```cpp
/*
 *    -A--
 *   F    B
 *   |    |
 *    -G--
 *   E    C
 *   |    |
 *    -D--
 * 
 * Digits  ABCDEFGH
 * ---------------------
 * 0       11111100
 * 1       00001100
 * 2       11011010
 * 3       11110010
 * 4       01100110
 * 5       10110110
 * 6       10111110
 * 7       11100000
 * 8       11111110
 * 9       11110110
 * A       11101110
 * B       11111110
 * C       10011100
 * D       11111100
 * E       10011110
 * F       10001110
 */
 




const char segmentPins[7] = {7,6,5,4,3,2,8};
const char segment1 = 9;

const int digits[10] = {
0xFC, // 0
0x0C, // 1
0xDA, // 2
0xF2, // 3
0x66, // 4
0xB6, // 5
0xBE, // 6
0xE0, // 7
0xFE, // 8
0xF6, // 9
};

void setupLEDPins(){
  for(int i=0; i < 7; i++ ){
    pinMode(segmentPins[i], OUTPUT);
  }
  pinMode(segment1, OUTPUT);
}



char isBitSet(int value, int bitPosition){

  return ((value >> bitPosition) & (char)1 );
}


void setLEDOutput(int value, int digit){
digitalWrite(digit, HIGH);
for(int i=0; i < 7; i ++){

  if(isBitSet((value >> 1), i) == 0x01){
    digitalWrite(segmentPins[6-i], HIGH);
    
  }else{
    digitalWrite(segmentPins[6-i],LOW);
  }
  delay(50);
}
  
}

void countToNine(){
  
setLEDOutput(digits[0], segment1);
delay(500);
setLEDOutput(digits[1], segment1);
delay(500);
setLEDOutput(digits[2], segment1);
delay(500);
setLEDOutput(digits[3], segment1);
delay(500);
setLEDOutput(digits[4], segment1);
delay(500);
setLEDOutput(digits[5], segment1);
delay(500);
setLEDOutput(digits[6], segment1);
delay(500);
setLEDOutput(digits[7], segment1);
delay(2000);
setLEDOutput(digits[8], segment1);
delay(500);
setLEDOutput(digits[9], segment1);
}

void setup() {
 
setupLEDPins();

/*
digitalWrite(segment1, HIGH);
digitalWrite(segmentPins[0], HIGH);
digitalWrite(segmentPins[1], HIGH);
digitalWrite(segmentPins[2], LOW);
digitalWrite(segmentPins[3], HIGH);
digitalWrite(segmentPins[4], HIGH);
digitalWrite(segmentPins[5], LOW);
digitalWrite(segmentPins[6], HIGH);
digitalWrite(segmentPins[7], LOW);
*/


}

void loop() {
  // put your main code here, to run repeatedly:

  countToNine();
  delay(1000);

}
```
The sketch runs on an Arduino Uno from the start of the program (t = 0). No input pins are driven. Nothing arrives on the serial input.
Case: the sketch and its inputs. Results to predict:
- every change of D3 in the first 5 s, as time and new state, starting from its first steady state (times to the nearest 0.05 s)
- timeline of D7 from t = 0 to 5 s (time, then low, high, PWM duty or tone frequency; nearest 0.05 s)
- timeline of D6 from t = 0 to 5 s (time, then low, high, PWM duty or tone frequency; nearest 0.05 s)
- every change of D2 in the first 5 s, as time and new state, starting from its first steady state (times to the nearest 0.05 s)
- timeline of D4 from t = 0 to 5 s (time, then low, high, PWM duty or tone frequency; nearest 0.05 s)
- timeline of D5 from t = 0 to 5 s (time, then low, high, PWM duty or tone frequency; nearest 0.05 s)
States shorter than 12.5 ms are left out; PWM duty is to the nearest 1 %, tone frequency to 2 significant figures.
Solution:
0 s low; 0.1 s high; 2.65 s low
0 s low; 0.3 s high; 1.15 s low; 2 s high; 3.7 s low; 4.55 s high
0 s low; 0.25 s high; 1.1 s low; 1.95 s high; 4.5 s low
0 s low; 0.05 s high; 1.75 s low; 3.45 s high
0 s low; 0.15 s high; 1 s low; 1.85 s high; 3.55 s low; 4.4 s high
0 s low; 0.2 s high; 1.05 s low; 2.75 s high
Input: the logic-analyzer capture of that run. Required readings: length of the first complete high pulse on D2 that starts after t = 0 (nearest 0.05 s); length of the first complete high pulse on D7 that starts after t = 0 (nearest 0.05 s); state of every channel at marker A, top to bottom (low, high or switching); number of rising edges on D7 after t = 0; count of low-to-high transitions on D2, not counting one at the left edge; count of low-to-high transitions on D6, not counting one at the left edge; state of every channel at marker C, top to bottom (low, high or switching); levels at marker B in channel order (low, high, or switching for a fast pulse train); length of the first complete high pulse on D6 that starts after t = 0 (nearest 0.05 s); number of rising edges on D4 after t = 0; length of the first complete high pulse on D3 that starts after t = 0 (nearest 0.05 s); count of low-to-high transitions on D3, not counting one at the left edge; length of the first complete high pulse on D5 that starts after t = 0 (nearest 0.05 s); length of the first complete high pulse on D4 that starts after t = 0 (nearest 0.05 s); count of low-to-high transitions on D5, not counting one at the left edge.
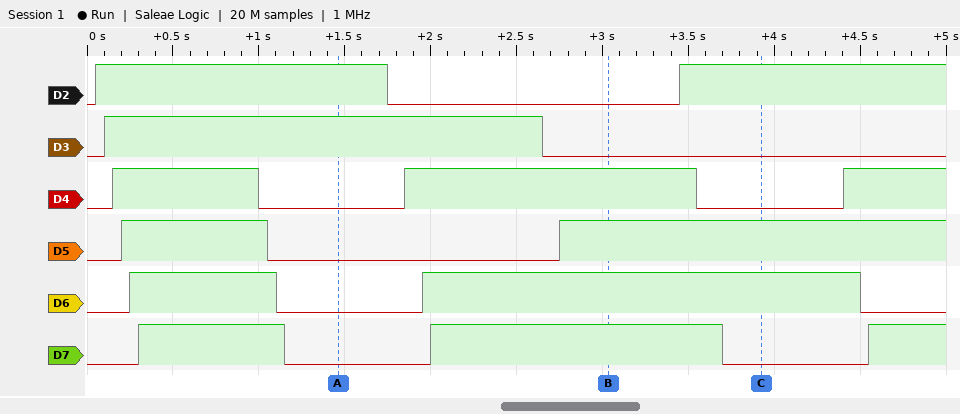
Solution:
1.70 s
0.85 s
D2 high, D3 high, D4 low, D5 low, D6 low, D7 low
3
2
2
D2 high, D3 low, D4 low, D5 high, D6 high, D7 low
D2 low, D3 low, D4 high, D5 high, D6 high, D7 high
0.85 s
3
2.55 s
1
0.85 s
0.85 s
2
